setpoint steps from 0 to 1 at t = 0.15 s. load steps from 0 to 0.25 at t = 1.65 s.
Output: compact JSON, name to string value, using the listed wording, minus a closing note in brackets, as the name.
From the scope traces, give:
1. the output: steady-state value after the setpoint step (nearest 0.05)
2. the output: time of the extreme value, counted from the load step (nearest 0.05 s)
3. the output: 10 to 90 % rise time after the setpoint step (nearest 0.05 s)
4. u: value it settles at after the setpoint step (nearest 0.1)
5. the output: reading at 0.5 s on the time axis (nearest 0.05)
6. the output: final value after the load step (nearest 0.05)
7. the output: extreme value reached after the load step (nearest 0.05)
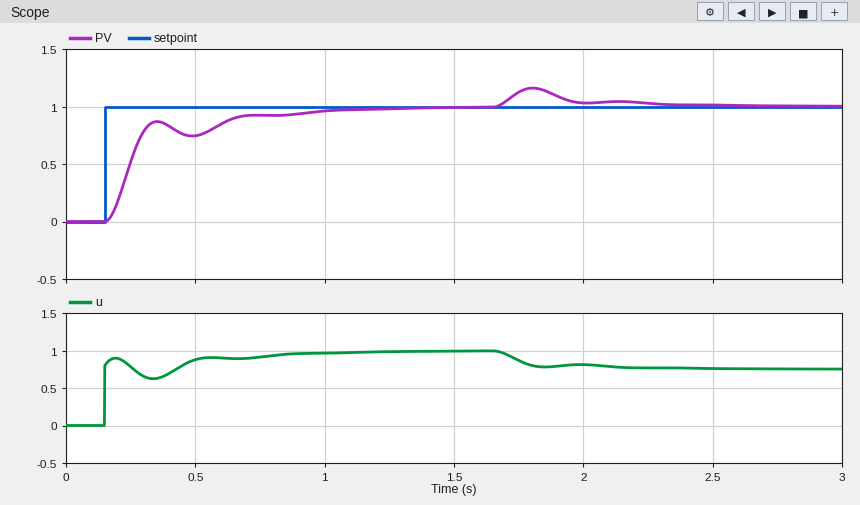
{"the output: steady-state value after the setpoint step": "1.00", "the output: time of the extreme value, counted from the load step": "0.15 s", "the output: 10 to 90 % rise time after the setpoint step": "0.45 s", "u: value it settles at after the setpoint step": "1.0", "the output: reading at 0.5 s on the time axis": "0.75", "the output: final value after the load step": "1.00", "the output: extreme value reached after the load step": "1.15"}
